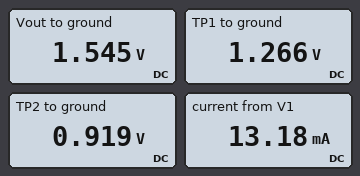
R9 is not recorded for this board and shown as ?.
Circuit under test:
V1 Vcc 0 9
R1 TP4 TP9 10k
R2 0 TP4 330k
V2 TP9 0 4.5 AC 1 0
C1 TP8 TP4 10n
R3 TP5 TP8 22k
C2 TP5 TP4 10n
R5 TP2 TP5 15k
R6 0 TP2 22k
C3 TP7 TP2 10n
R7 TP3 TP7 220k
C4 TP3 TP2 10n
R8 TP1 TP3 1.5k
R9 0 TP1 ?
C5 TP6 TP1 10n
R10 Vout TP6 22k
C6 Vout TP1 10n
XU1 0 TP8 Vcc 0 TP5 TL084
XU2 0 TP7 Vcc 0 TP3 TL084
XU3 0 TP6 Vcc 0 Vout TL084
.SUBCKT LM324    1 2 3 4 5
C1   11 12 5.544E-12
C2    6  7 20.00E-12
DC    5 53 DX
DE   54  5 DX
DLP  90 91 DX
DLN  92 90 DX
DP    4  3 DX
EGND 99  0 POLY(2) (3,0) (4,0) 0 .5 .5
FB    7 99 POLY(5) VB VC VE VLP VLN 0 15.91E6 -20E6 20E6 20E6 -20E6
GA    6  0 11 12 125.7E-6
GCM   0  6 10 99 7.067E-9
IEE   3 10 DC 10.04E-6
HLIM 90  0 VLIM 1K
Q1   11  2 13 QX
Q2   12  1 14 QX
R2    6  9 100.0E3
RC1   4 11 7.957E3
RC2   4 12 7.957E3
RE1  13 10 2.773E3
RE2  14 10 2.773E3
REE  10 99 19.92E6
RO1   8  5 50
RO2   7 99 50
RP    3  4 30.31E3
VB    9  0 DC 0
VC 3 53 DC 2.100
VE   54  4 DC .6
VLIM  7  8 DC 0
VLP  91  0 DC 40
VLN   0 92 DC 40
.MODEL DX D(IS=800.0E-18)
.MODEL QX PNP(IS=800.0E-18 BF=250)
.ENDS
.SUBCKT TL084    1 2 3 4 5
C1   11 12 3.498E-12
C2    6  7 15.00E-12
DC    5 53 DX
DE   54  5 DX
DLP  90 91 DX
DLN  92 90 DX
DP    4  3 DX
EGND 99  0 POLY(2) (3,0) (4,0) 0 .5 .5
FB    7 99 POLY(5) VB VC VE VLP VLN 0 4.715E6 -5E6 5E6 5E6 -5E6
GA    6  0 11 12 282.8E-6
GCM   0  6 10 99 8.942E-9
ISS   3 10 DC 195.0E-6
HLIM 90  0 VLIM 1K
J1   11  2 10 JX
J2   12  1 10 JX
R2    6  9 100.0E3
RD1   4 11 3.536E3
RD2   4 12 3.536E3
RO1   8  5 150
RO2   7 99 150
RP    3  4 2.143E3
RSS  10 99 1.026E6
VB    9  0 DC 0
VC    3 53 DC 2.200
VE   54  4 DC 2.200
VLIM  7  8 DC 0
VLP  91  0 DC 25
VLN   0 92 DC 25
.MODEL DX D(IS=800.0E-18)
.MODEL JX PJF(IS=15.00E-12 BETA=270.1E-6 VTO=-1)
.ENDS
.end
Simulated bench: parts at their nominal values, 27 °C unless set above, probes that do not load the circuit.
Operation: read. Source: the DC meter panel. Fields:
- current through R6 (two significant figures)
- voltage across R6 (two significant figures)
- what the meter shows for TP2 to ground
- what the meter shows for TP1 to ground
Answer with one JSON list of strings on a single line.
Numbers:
["42 µA", "920 mV", "0.919 V", "1.266 V"]
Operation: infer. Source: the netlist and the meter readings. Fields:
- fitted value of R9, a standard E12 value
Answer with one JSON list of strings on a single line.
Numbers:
["6.8 kΩ"]
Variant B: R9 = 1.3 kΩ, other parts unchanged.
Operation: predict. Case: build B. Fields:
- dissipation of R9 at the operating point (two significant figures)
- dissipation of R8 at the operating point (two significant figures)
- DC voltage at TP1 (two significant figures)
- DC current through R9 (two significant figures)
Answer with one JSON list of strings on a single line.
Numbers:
["400 µW", "460 µW", "720 mV", "550 µA"]
